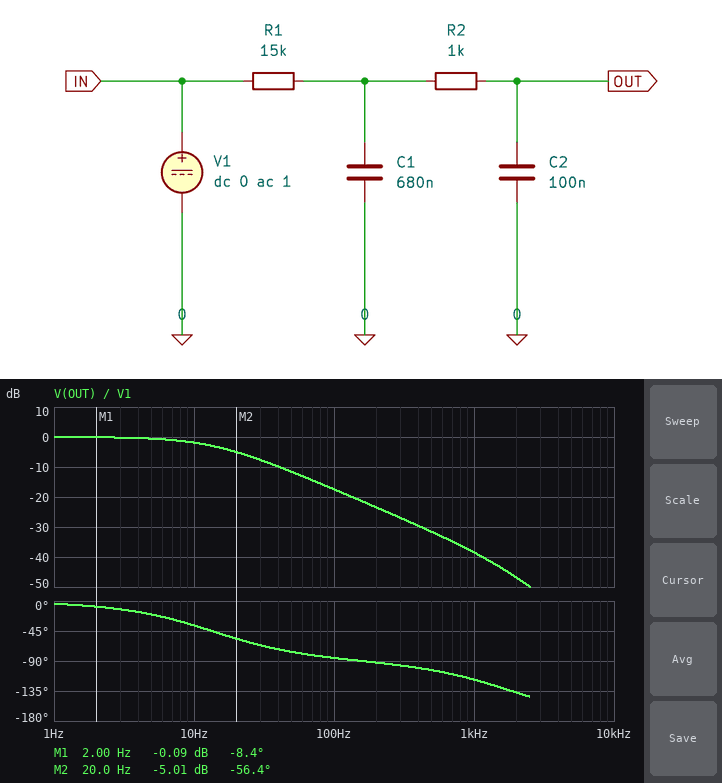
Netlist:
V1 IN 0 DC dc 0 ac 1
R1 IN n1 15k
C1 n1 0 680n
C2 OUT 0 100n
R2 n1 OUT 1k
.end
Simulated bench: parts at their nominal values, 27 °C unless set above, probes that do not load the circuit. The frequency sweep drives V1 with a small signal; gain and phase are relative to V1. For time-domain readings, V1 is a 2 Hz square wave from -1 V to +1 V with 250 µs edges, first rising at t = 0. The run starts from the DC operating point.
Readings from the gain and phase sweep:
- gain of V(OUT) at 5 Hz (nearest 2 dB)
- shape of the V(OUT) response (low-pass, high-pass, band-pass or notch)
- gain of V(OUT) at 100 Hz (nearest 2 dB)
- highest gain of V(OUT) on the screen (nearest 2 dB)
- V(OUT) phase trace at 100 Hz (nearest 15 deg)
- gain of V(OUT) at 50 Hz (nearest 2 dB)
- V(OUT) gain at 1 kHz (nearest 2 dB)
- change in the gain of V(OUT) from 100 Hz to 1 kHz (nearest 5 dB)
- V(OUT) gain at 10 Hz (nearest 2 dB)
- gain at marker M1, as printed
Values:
0 dB
low-pass
-18 dB
0 dB
-90 deg
-12 dB
-38 dB
-20 dB
-2 dB
-0.09 dB
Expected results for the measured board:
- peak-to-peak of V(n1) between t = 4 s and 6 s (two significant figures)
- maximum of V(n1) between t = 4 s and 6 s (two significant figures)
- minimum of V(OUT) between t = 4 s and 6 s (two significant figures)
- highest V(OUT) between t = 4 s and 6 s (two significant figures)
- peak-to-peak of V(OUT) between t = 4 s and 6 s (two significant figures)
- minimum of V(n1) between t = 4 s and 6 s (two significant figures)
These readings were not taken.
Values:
2.0 V
1.0 V
-1.0 V
1.0 V
2.0 V
-1.0 V
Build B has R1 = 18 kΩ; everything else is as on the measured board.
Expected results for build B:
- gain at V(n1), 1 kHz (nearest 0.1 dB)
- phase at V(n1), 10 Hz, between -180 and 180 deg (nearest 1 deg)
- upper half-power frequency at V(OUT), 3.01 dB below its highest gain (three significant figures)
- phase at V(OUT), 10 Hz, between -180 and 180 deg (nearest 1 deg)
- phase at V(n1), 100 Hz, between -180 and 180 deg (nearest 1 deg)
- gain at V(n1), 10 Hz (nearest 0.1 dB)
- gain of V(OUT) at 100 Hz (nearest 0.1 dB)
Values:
-38.6 dB
-41 deg
11.3 Hz
-42 deg
-83 deg
-2.5 dB
-19.0 dB
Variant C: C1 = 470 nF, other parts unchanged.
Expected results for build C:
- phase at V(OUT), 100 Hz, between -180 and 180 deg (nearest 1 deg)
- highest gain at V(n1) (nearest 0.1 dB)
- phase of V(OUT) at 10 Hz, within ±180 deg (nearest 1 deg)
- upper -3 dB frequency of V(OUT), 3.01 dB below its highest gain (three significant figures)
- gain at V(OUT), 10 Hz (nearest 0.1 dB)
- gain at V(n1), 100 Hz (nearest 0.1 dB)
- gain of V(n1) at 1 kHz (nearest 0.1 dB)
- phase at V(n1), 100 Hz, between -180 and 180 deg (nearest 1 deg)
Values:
-82 deg
0 dB
-29 deg
18.6 Hz
-1.1 dB
-14.8 dB
-34.2 dB
-79 deg
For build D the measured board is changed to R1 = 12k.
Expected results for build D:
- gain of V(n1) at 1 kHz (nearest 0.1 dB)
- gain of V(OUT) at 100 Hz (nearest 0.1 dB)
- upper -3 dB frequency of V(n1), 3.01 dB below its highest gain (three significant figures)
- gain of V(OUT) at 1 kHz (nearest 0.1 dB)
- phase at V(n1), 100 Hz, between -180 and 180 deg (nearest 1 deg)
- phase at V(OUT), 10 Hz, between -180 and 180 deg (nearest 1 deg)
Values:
-35.1 dB
-15.5 dB
17.0 Hz
-36.5 dB
-80 deg
-31 deg
